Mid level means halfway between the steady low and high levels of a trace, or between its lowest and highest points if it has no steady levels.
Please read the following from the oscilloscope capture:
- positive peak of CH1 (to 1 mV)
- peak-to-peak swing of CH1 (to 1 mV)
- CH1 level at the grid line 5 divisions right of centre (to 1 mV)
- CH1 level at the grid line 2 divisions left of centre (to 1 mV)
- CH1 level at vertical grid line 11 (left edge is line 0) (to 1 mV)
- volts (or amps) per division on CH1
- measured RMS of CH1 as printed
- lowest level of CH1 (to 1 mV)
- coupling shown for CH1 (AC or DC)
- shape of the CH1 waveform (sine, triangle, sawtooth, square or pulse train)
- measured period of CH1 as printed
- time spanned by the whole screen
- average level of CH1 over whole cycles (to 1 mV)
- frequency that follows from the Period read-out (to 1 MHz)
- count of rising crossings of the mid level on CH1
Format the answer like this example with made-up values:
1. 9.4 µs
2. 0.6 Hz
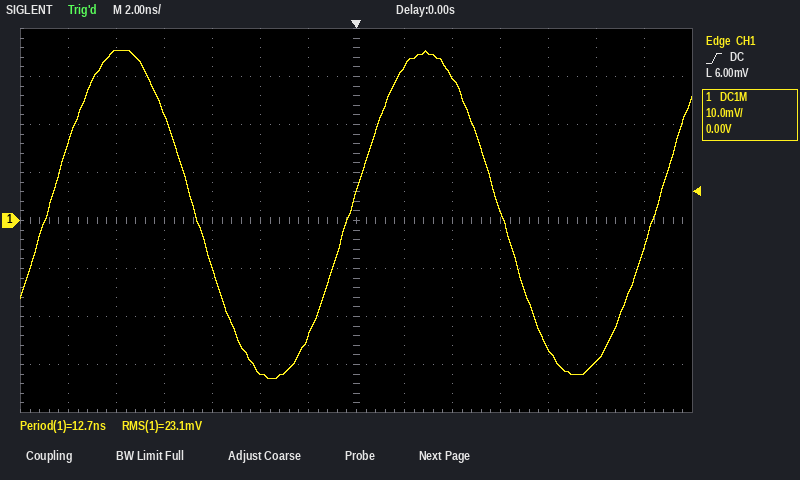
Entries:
1. 35 mV
2. 68 mV
3. -29 mV
4. -32 mV
5. -27 mV
6. 10 mV
7. 23.1 mV
8. -33 mV
9. DC
10. sine
11. 12.7 ns
12. 28 ns
13. 1 mV
14. 79 MHz
15. 3
